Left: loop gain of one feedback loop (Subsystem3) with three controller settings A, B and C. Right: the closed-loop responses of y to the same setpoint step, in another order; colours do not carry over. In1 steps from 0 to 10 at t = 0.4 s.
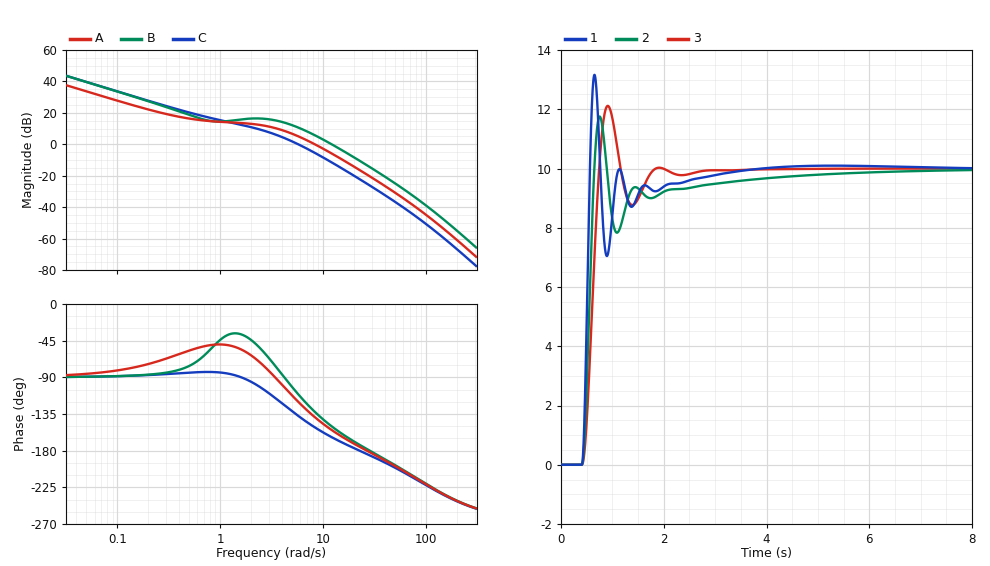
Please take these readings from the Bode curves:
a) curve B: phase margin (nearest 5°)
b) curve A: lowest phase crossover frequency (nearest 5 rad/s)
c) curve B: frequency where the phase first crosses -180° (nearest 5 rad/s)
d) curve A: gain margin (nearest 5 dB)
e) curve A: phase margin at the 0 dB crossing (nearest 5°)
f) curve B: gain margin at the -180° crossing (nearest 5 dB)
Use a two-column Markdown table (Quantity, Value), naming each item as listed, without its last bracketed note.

| Quantity | Value |
|---|---|
| curve B: phase margin | 30° |
| curve A: lowest phase crossover frequency | 25 rad/s |
| curve B: frequency where the phase first crosses -180° | 30 rad/s |
| curve A: gain margin | 20 dB |
| curve A: phase margin at the 0 dB crossing | 40° |
| curve B: gain margin at the -180° crossing | 15 dB |
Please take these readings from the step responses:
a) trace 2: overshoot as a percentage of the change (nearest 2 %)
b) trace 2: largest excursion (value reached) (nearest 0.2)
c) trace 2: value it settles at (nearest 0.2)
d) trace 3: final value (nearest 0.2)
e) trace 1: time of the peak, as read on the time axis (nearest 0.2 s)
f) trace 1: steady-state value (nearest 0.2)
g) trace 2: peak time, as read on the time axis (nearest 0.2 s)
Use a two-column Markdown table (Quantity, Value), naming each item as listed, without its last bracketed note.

| Quantity | Value |
|---|---|
| trace 2: overshoot as a percentage of the change | 18 % |
| trace 2: largest excursion (value reached) | 11.8 |
| trace 2: value it settles at | 10.0 |
| trace 3: final value | 10.0 |
| trace 1: time of the peak, as read on the time axis | 0.6 s |
| trace 1: steady-state value | 10.0 |
| trace 2: peak time, as read on the time axis | 0.8 s |
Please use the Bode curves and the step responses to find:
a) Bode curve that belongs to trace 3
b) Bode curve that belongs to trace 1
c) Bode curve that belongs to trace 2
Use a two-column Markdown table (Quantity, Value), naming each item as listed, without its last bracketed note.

| Quantity | Value |
|---|---|
| Bode curve that belongs to trace 3 | C |
| Bode curve that belongs to trace 1 | B |
| Bode curve that belongs to trace 2 | A |
